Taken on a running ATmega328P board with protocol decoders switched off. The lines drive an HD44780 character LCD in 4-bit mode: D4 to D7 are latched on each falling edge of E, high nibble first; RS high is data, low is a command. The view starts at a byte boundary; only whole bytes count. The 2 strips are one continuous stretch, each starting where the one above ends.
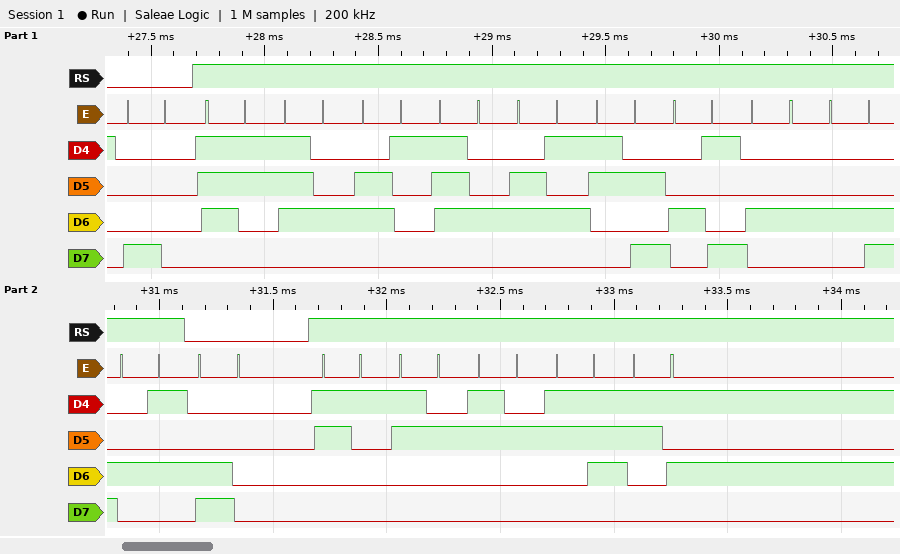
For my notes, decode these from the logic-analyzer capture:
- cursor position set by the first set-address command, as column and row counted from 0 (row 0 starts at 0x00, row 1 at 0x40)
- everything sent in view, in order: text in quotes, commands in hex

column 0, row 0
0x80 "state:IDLE" 0xC0 "12275"
